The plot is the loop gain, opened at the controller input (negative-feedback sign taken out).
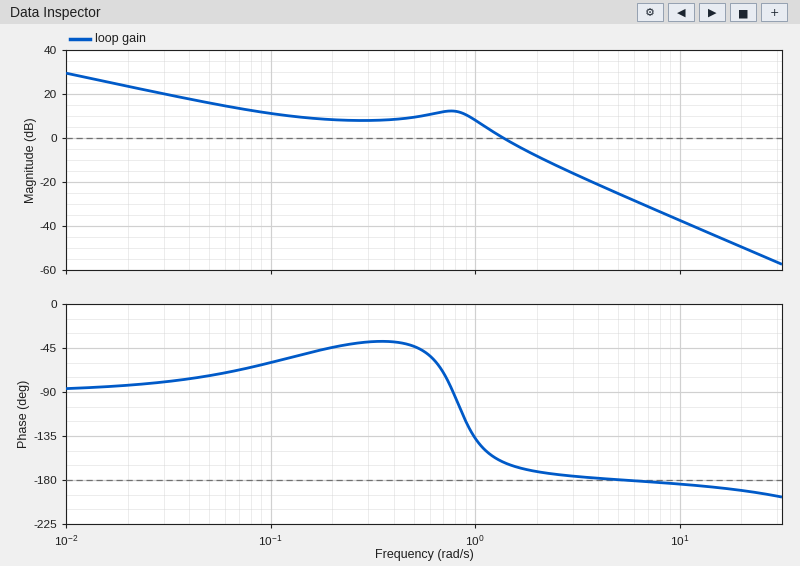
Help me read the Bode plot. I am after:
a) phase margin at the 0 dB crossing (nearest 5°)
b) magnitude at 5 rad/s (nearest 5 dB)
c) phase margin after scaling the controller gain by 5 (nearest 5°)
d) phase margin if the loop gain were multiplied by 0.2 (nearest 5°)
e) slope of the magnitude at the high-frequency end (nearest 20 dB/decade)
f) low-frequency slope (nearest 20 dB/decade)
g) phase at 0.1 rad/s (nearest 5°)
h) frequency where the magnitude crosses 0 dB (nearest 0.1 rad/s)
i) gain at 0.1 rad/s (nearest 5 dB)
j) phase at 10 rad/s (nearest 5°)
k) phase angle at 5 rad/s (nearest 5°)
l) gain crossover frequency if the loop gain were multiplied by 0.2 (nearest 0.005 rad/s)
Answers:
20°
-25 dB
5°
110°
-40 dB/decade
-20 dB/decade
-60°
1.4 rad/s
10 dB
-185°
-180°
0.065 rad/s
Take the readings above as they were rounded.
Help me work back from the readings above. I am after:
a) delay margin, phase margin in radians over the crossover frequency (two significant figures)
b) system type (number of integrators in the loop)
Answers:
0.25 s
1
